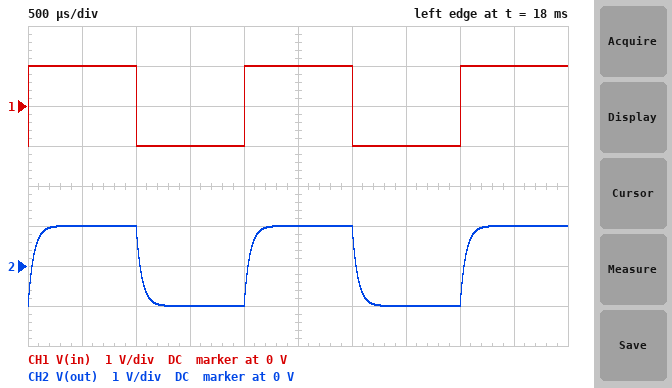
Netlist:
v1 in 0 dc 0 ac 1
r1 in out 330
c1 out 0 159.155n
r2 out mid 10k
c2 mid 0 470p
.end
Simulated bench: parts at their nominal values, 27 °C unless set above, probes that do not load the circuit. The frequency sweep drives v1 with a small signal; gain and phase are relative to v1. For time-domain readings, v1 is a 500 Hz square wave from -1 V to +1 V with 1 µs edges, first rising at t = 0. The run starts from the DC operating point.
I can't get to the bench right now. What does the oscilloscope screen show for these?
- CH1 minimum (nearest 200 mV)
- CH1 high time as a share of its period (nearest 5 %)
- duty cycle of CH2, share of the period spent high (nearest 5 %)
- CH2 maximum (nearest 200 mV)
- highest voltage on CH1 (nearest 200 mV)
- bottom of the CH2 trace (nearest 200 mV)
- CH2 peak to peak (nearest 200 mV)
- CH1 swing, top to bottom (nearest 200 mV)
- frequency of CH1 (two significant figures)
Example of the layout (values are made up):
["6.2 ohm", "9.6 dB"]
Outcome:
["-1.0 V", "50 %", "50 %", "1.0 V", "1.0 V", "-1.0 V", "2.0 V", "2.0 V", "500 Hz"]
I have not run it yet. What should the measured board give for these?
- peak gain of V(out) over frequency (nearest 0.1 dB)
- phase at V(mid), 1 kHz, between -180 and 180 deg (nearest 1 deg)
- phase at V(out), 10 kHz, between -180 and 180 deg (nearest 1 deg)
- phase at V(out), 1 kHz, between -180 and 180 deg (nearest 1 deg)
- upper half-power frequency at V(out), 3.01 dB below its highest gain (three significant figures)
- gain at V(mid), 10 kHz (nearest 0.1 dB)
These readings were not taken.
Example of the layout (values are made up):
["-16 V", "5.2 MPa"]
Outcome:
["0 dB", "-20 deg", "-73 deg", "-18 deg", "3.02 kHz", "-11.1 dB"]
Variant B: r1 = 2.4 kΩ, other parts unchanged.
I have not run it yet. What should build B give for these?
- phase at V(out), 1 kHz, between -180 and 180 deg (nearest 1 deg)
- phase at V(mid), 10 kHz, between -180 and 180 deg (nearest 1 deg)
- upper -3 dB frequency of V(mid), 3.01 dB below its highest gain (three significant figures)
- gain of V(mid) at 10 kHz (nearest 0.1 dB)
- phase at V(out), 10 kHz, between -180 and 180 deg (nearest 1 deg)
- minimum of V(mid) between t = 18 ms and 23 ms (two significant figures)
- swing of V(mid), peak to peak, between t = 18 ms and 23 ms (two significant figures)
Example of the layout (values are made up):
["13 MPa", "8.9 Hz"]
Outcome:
["-67 deg", "-104 deg", "415 Hz", "-28.0 dB", "-88 deg", "-860 mV", "1.7 V"]
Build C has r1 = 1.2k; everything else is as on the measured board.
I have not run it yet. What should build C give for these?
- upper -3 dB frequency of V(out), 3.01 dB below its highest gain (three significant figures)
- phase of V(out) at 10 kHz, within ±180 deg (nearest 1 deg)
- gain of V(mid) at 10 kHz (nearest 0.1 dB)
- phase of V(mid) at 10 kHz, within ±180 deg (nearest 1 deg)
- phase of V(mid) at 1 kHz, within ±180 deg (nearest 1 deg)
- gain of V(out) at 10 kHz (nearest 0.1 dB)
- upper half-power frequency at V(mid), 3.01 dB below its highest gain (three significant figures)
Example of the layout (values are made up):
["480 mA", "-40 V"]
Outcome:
["831 Hz", "-85 deg", "-22.0 dB", "-102 deg", "-52 deg", "-21.6 dB", "830 Hz"]
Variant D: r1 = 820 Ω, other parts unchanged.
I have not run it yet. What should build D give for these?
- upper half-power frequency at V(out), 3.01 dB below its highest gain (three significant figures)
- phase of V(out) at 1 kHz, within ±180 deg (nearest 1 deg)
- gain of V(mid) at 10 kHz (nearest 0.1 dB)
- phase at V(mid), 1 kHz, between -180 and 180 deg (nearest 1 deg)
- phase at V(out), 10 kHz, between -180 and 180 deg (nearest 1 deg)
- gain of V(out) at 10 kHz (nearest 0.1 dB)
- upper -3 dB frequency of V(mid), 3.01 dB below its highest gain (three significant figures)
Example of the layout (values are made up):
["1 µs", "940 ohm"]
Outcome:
["1.22 kHz", "-39 deg", "-18.7 dB", "-41 deg", "-83 deg", "-18.4 dB", "1.21 kHz"]
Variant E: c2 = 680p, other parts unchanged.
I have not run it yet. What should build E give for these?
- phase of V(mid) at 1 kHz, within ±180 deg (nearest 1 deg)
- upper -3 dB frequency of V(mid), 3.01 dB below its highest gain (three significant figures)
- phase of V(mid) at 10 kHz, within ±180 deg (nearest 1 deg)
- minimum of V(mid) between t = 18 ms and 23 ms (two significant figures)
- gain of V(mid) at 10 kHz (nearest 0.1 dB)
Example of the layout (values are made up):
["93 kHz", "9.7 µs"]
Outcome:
["-21 deg", "2.97 kHz", "-96 deg", "-1.0 V", "-11.5 dB"]
